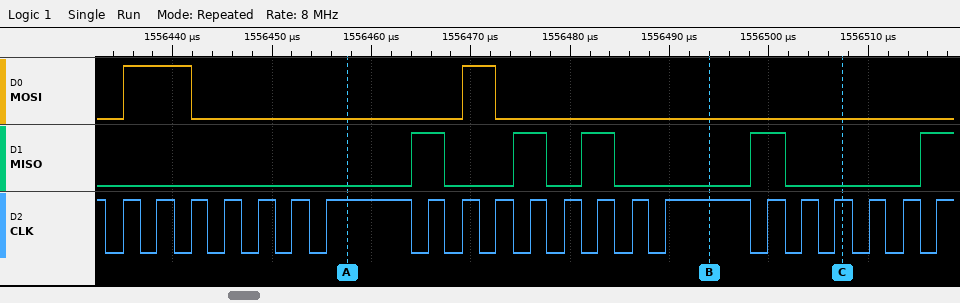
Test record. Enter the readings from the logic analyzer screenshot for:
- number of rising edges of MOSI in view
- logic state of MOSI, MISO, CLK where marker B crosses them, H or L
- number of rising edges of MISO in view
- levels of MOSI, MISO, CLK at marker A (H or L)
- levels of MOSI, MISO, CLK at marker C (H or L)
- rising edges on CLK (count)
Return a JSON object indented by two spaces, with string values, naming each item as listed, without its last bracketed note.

{
  "number of rising edges of MOSI in view": "2",
  "logic state of MOSI, MISO, CLK where marker B crosses them, H or L": "MOSI=L, MISO=L, CLK=H",
  "number of rising edges of MISO in view": "5",
  "levels of MOSI, MISO, CLK at marker A": "MOSI=L, MISO=L, CLK=H",
  "levels of MOSI, MISO, CLK at marker C": "MOSI=L, MISO=L, CLK=H",
  "rising edges on CLK": "21"
}
